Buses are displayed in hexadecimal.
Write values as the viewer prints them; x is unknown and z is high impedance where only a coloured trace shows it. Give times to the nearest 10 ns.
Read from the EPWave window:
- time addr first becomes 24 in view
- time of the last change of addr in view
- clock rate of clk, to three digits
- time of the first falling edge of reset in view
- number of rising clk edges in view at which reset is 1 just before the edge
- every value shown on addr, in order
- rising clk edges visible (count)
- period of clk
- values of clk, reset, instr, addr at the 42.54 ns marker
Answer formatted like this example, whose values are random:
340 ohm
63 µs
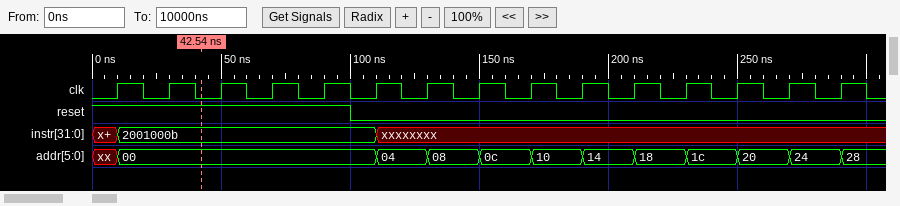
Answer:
270 ns
290 ns
50.0 MHz
100 ns
5
xx, 00, 04, 08, 0c, 10, 14, 18, 1c, 20, 24, 28
15
20 ns
clk=0, reset=1, instr=2001000b, addr=00
